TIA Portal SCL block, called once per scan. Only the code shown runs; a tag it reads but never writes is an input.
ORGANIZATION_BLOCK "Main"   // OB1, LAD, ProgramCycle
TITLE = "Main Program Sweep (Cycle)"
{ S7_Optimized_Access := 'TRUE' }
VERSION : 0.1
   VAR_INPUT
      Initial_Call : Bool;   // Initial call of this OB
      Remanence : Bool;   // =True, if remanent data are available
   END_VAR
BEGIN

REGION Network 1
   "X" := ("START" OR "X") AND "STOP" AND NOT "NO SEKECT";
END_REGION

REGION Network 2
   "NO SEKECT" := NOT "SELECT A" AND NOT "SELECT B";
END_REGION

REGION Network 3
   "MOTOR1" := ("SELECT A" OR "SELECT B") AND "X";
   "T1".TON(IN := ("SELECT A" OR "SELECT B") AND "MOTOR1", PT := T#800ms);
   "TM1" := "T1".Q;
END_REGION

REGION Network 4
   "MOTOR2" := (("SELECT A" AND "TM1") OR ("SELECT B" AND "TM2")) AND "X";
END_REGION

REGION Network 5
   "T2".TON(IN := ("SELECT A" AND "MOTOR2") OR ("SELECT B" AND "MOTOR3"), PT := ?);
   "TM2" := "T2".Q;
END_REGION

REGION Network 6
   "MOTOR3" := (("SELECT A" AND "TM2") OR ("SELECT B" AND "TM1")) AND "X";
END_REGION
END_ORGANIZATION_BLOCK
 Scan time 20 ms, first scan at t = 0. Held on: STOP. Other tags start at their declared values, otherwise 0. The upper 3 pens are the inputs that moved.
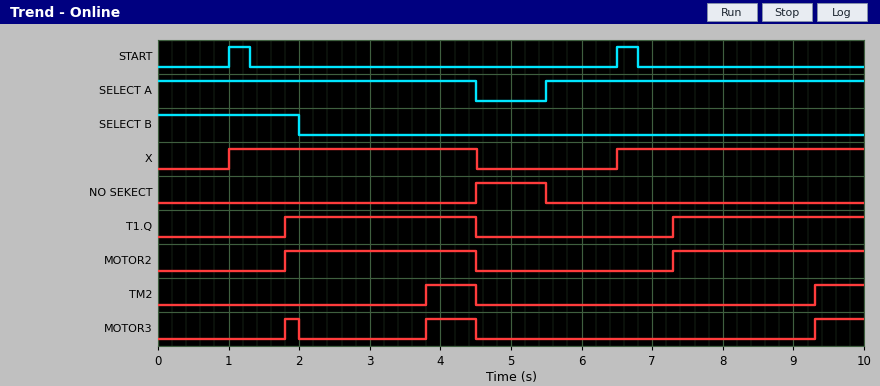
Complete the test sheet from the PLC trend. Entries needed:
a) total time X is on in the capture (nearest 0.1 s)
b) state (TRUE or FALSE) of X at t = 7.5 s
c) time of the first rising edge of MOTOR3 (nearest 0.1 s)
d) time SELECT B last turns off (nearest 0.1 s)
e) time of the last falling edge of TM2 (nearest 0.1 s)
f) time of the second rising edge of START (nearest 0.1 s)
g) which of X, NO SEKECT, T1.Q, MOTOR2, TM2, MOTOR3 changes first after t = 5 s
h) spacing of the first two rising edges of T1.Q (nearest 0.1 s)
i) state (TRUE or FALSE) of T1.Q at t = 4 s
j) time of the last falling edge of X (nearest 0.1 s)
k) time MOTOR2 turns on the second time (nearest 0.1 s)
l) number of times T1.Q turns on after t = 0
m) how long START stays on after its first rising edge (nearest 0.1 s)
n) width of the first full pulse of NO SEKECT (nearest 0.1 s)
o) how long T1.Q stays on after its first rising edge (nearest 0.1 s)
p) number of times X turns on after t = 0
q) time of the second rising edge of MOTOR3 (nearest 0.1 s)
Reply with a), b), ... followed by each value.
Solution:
a) 7.0 s
b) TRUE
c) 1.8 s
d) 2.0 s
e) 4.5 s
f) 6.5 s
g) NO SEKECT
h) 5.5 s
i) TRUE
j) 4.5 s
k) 7.3 s
l) 2
m) 0.3 s
n) 1.0 s
o) 2.7 s
p) 2
q) 3.8 s
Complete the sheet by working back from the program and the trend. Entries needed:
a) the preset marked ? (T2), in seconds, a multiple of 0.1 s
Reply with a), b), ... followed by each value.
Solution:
a) 2.0 s
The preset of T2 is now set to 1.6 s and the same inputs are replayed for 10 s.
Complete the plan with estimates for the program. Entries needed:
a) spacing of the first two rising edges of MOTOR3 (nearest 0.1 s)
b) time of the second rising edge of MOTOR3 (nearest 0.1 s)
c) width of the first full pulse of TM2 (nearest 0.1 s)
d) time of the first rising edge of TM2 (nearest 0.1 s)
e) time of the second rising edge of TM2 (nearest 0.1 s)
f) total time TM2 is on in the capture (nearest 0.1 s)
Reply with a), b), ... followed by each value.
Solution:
a) 1.6 s
b) 3.4 s
c) 1.1 s
d) 3.4 s
e) 8.9 s
f) 2.2 s
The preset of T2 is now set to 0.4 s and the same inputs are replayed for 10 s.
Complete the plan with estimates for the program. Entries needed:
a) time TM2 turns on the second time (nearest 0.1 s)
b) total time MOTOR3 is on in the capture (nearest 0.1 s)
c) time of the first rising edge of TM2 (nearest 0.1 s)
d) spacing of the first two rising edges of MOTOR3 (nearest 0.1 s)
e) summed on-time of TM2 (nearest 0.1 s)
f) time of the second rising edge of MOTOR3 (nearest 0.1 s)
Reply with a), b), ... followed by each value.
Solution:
a) 7.7 s
b) 4.8 s
c) 2.2 s
d) 0.4 s
e) 4.6 s
f) 2.2 s
